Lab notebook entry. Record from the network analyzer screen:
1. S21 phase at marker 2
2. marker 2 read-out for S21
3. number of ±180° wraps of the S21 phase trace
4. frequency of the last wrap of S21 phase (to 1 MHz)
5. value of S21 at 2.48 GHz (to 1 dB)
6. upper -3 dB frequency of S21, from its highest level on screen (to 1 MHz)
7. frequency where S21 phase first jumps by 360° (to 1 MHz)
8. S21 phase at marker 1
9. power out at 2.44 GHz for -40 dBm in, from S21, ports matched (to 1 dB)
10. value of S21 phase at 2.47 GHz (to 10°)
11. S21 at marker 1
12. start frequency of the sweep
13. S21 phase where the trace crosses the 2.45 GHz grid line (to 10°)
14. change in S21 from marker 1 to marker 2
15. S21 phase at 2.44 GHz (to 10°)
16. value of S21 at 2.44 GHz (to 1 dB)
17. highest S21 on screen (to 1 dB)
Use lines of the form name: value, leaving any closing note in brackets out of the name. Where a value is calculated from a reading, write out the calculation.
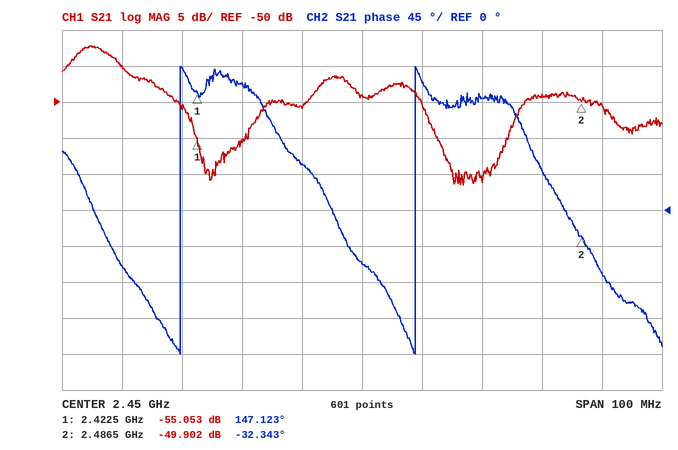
S21 phase at marker 2: -32.343°
marker 2 read-out for S21: -49.902 dB
number of ±180° wraps of the S21 phase trace: 2
frequency of the last wrap of S21 phase: 2.459 GHz
value of S21 at 2.48 GHz: -49 dB
upper -3 dB frequency of S21, from its highest level on screen: 2.410 GHz
frequency where S21 phase first jumps by 360°: 2.420 GHz
S21 phase at marker 1: 147.123°
power out at 2.44 GHz for -40 dBm in, from S21, ports matched: -40 dBm + (-51 dB) = -91 dBm
value of S21 phase at 2.47 GHz: 140°
S21 at marker 1: -55.053 dB
start frequency of the sweep: 2.4 GHz
S21 phase where the trace crosses the 2.45 GHz grid line: -70°
change in S21 from marker 1 to marker 2: -49.902 − (-55.053) = 5.151 dB
S21 phase at 2.44 GHz: 60°
value of S21 at 2.44 GHz: -51 dB
highest S21 on screen: -42 dB
